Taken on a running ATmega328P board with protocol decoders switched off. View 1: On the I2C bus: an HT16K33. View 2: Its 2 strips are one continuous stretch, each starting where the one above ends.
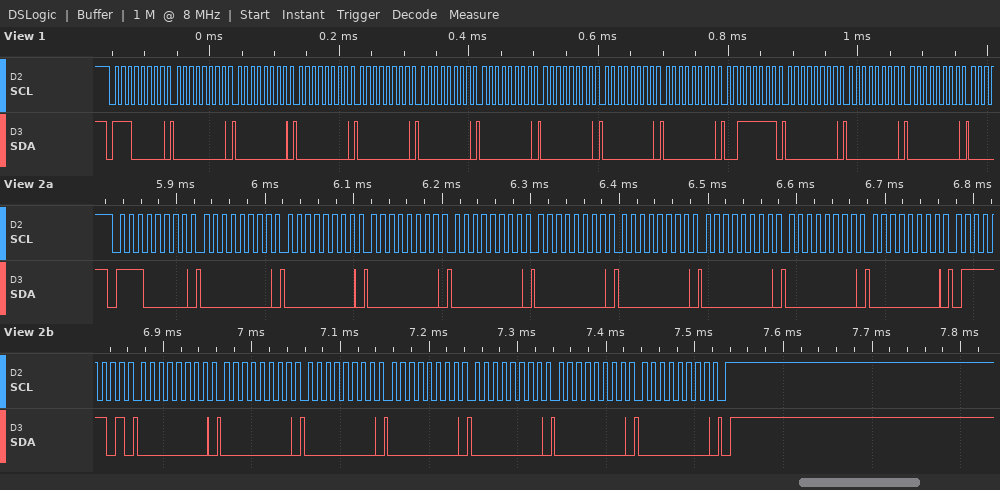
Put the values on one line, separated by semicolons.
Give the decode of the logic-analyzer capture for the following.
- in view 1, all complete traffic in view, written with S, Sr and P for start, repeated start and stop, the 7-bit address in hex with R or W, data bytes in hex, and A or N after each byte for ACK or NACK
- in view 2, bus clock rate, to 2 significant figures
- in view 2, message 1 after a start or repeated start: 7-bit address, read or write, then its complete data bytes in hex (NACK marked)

S 70W A 00 A 00 A 00 A 00 A 00 A 00 A 00 A 00 A 00 A 3F A 00 A 00 A 00 A; 100 kHz; 0x70 write: 00 00 00 00 00 00 00 00 00 7D 00 00 00 00 00 00 00
